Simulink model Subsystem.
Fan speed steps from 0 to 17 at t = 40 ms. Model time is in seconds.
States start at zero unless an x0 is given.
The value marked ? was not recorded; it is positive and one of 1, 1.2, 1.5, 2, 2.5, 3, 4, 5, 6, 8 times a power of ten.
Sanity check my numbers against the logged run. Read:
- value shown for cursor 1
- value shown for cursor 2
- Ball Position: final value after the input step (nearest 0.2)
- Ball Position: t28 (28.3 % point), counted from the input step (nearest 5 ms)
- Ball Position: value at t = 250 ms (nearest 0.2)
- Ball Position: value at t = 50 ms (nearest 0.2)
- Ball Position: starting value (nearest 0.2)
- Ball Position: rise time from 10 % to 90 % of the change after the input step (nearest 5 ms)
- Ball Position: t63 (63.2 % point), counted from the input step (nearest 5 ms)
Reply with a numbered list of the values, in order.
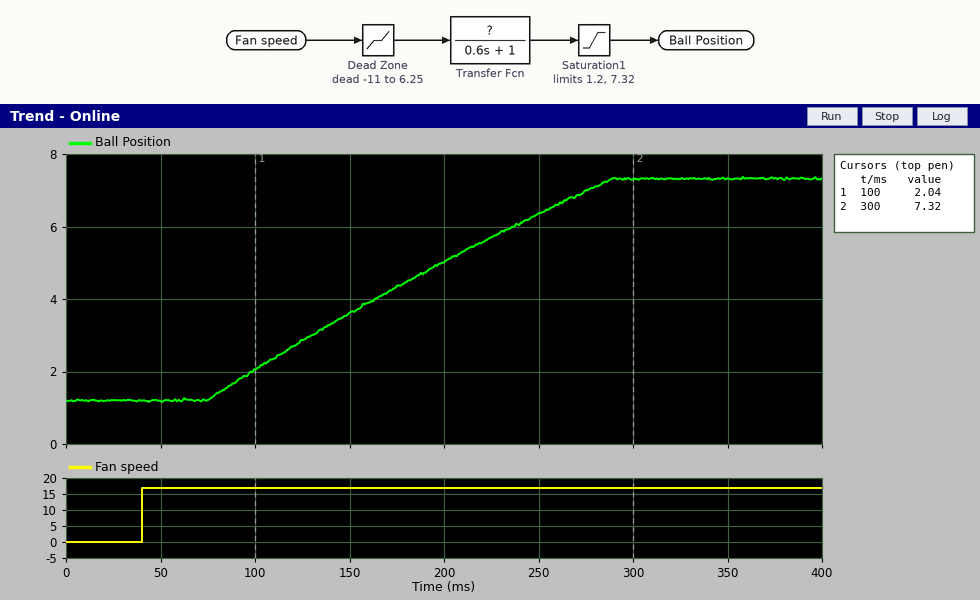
1. 2.04
2. 7.32
3. 7.4
4. 90 ms
5. 6.4
6. 1.2
7. 1.2
8. 170 ms
9. 160 ms
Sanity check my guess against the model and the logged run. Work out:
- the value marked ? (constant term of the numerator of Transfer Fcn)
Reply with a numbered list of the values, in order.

1. 2
